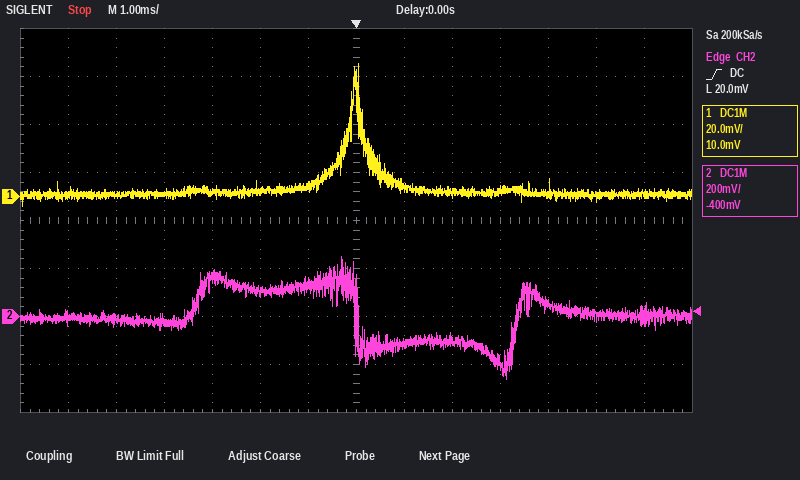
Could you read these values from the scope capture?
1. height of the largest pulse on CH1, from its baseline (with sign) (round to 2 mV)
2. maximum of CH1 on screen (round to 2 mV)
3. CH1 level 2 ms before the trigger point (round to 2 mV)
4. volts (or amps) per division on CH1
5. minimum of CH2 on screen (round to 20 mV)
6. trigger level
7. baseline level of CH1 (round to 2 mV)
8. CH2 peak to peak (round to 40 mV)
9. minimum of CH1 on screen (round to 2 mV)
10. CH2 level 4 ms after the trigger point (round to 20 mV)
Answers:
+54 mV
56 mV
2 mV
20 mV
-260 mV
20.0 mV
2 mV
520 mV
-4 mV
60 mV
